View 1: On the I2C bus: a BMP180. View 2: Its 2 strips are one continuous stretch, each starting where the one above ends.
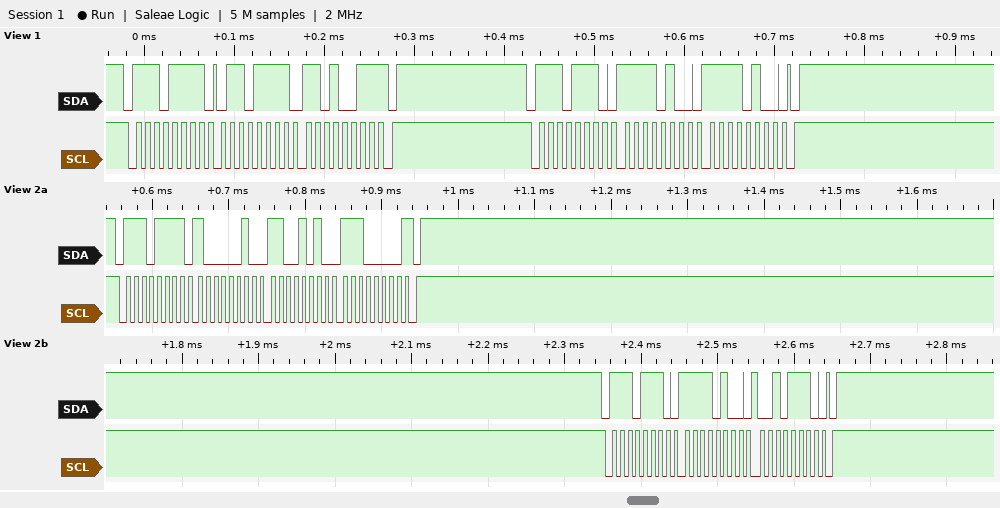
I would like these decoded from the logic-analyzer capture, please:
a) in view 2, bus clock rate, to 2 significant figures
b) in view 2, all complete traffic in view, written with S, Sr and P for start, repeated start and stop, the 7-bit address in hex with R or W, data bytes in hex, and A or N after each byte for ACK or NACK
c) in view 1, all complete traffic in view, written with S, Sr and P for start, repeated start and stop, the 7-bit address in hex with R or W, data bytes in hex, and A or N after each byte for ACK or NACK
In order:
100 kHz
S 77R A 82 A CA A E0 N P S 77W A F4 A 2E A P
S 77R A 6F A D3 N P S 77W A F4 A F4 A P
